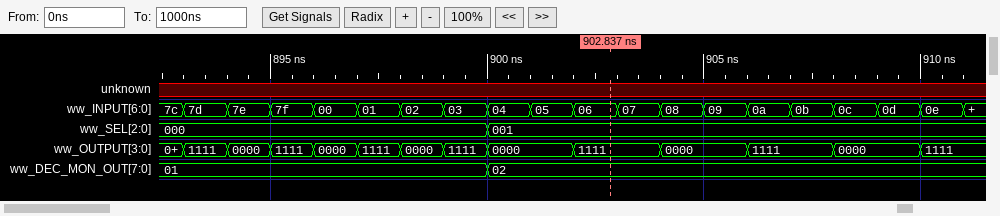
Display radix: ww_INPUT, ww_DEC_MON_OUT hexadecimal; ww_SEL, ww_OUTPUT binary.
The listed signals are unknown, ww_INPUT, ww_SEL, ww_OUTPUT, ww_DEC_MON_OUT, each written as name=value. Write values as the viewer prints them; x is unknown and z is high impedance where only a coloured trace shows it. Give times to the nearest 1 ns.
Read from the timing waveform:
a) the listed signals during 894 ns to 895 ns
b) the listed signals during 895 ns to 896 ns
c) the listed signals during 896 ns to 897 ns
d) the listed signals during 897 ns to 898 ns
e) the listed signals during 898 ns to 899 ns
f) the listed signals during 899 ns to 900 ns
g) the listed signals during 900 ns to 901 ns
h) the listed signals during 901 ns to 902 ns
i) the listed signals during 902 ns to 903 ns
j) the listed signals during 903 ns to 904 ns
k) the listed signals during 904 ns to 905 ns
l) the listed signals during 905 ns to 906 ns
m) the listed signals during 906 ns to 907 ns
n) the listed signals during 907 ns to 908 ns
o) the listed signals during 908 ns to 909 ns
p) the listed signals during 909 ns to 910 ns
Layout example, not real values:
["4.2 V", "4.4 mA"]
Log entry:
["unknown=x, ww_INPUT=7e, ww_SEL=000, ww_OUTPUT=0000, ww_DEC_MON_OUT=01", "unknown=x, ww_INPUT=7f, ww_SEL=000, ww_OUTPUT=1111, ww_DEC_MON_OUT=01", "unknown=x, ww_INPUT=00, ww_SEL=000, ww_OUTPUT=0000, ww_DEC_MON_OUT=01", "unknown=x, ww_INPUT=01, ww_SEL=000, ww_OUTPUT=1111, ww_DEC_MON_OUT=01", "unknown=x, ww_INPUT=02, ww_SEL=000, ww_OUTPUT=0000, ww_DEC_MON_OUT=01", "unknown=x, ww_INPUT=03, ww_SEL=000, ww_OUTPUT=1111, ww_DEC_MON_OUT=01", "unknown=x, ww_INPUT=04, ww_SEL=001, ww_OUTPUT=0000, ww_DEC_MON_OUT=02", "unknown=x, ww_INPUT=05, ww_SEL=001, ww_OUTPUT=0000, ww_DEC_MON_OUT=02", "unknown=x, ww_INPUT=06, ww_SEL=001, ww_OUTPUT=1111, ww_DEC_MON_OUT=02", "unknown=x, ww_INPUT=07, ww_SEL=001, ww_OUTPUT=1111, ww_DEC_MON_OUT=02", "unknown=x, ww_INPUT=08, ww_SEL=001, ww_OUTPUT=0000, ww_DEC_MON_OUT=02", "unknown=x, ww_INPUT=09, ww_SEL=001, ww_OUTPUT=0000, ww_DEC_MON_OUT=02", "unknown=x, ww_INPUT=0a, ww_SEL=001, ww_OUTPUT=1111, ww_DEC_MON_OUT=02", "unknown=x, ww_INPUT=0b, ww_SEL=001, ww_OUTPUT=1111, ww_DEC_MON_OUT=02", "unknown=x, ww_INPUT=0c, ww_SEL=001, ww_OUTPUT=0000, ww_DEC_MON_OUT=02", "unknown=x, ww_INPUT=0d, ww_SEL=001, ww_OUTPUT=0000, ww_DEC_MON_OUT=02"]
